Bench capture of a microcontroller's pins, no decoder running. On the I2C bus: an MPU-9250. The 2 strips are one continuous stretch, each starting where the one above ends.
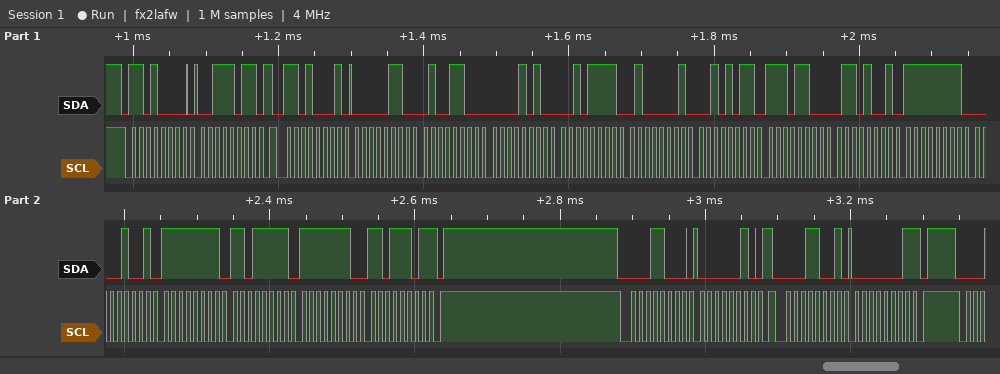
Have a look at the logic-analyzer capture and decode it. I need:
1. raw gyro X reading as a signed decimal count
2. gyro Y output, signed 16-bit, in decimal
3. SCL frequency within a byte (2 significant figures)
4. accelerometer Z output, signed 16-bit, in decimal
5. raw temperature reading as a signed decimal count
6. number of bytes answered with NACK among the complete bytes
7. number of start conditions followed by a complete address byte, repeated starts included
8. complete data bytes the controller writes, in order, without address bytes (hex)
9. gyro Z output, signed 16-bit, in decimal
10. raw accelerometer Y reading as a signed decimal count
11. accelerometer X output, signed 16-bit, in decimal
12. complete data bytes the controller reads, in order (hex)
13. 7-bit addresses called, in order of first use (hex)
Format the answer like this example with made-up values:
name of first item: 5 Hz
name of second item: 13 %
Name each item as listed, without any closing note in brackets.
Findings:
raw gyro X reading as a signed decimal count: -247
gyro Y output, signed 16-bit, in decimal: -33
SCL frequency within a byte: 100 kHz
accelerometer Z output, signed 16-bit, in decimal: 16683
raw temperature reading as a signed decimal count: -5015
number of bytes answered with NACK among the complete bytes: 2
number of start conditions followed by a complete address byte, repeated starts included: 4
complete data bytes the controller writes, in order, without address bytes: 3B 02
gyro Z output, signed 16-bit, in decimal: -291
raw accelerometer Y reading as a signed decimal count: 2607
accelerometer X output, signed 16-bit, in decimal: 1612
complete data bytes the controller reads, in order: 06 4C 0A 2F 41 2B EC 69 FF 09 FF DF FE DD 01
7-bit addresses called, in order of first use: 0x68 0x0C
